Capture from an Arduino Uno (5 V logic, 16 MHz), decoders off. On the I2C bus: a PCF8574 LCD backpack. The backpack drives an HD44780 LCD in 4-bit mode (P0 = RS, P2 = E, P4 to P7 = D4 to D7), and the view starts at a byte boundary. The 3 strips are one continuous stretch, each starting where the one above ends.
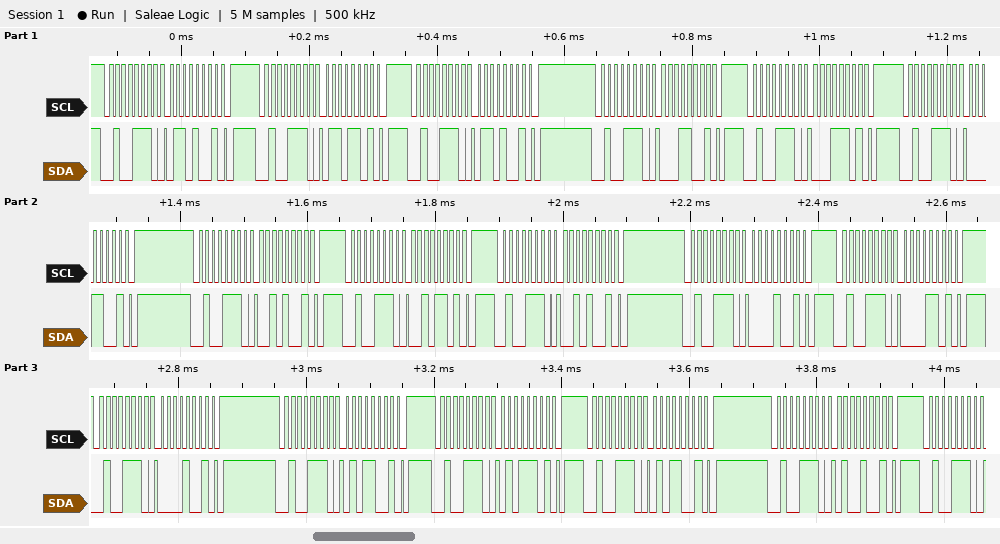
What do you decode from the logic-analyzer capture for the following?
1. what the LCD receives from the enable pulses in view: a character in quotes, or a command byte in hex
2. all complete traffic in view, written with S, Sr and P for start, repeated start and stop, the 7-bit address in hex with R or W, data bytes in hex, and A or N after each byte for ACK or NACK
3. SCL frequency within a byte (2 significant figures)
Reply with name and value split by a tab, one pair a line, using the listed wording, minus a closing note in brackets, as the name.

what the LCD receives from the enable pulses in view: a character in quotes, or a command byte in hex	'a' ' '
all complete traffic in view, written with S, Sr and P for start, repeated start and stop, the 7-bit address in hex with R or W, data bytes in hex, and A or N after each byte for ACK or NACK	S 27W A 69 A P S 27W A 6D A P S 27W A 69 A P S 27W A 19 A P S 27W A 1D A P S 27W A 19 A P S 27W A 29 A P S 27W A 2D A P S 27W A 29 A P S 27W A 09 A P S 27W A 0D A P S 27W A 09 A P S 27W A 59 A P S 27W A 5D A P S 27W A 59 A P S 27W A 49 A P S 27W A
SCL frequency within a byte	100 kHz
